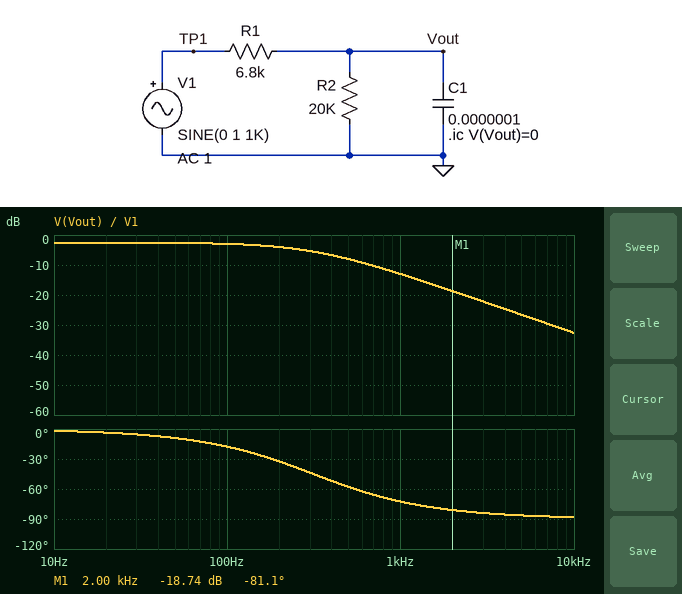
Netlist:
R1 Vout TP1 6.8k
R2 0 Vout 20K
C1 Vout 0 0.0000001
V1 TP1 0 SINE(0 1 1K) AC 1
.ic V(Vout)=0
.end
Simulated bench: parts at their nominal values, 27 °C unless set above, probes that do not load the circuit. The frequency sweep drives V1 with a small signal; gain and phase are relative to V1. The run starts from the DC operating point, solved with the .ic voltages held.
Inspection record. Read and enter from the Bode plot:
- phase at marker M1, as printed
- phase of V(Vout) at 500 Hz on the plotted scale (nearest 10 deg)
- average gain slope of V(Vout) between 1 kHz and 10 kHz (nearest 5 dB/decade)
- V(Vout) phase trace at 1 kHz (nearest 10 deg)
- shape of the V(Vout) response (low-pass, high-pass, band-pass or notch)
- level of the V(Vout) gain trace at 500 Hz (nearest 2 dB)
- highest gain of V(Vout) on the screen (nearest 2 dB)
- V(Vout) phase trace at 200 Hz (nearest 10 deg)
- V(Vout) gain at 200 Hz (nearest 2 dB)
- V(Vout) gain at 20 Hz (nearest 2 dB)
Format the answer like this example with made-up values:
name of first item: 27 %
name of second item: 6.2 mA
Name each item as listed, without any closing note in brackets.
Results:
phase at marker M1, as printed: -81.1 deg
phase of V(Vout) at 500 Hz on the plotted scale: -60 deg
average gain slope of V(Vout) between 1 kHz and 10 kHz: -20 dB/decade
V(Vout) phase trace at 1 kHz: -70 deg
shape of the V(Vout) response: low-pass
level of the V(Vout) gain trace at 500 Hz: -8 dB
highest gain of V(Vout) on the screen: -2 dB
V(Vout) phase trace at 200 Hz: -30 deg
V(Vout) gain at 200 Hz: -4 dB
V(Vout) gain at 20 Hz: -2 dB
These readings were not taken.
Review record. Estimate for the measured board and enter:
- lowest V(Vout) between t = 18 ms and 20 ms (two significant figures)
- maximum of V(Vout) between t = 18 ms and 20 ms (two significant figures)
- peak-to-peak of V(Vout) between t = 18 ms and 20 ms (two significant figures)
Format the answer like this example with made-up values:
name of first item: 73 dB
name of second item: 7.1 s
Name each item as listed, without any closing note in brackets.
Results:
lowest V(Vout) between t = 18 ms and 20 ms: -220 mV
maximum of V(Vout) between t = 18 ms and 20 ms: 220 mV
peak-to-peak of V(Vout) between t = 18 ms and 20 ms: 450 mV
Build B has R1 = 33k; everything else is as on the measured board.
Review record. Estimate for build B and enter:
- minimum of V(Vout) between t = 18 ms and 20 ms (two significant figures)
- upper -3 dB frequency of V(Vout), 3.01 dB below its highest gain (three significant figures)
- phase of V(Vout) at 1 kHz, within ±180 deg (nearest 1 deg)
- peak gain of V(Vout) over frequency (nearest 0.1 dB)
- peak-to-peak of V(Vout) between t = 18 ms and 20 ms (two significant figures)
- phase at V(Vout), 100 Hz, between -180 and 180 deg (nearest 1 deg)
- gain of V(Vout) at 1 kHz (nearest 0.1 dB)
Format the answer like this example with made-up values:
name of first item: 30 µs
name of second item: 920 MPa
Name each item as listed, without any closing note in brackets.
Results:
minimum of V(Vout) between t = 18 ms and 20 ms: -48 mV
upper -3 dB frequency of V(Vout), 3.01 dB below its highest gain: 128 Hz
phase of V(Vout) at 1 kHz, within ±180 deg: -83 deg
peak gain of V(Vout) over frequency: -8.5 dB
peak-to-peak of V(Vout) between t = 18 ms and 20 ms: 96 mV
phase at V(Vout), 100 Hz, between -180 and 180 deg: -38 deg
gain of V(Vout) at 1 kHz: -26.4 dB
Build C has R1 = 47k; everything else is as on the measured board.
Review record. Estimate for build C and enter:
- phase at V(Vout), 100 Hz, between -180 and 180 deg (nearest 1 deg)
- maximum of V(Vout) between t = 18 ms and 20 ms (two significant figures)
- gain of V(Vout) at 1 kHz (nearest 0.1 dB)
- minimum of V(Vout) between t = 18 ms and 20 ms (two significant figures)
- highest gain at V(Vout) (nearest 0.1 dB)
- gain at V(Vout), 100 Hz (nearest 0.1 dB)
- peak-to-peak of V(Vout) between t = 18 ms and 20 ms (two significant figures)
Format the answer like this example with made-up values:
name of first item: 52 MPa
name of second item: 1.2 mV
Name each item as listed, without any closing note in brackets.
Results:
phase at V(Vout), 100 Hz, between -180 and 180 deg: -41 deg
maximum of V(Vout) between t = 18 ms and 20 ms: 34 mV
gain of V(Vout) at 1 kHz: -29.5 dB
minimum of V(Vout) between t = 18 ms and 20 ms: -34 mV
highest gain at V(Vout): -10.5 dB
gain at V(Vout), 100 Hz: -13.0 dB
peak-to-peak of V(Vout) between t = 18 ms and 20 ms: 67 mV
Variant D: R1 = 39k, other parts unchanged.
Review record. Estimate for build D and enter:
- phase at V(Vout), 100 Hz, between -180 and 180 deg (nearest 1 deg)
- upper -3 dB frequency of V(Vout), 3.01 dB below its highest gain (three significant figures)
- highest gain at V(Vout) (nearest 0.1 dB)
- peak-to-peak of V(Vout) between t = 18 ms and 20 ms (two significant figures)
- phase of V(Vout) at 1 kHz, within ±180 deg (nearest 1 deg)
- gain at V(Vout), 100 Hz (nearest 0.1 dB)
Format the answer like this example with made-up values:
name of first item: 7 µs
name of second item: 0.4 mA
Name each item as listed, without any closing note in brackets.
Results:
phase at V(Vout), 100 Hz, between -180 and 180 deg: -40 deg
upper -3 dB frequency of V(Vout), 3.01 dB below its highest gain: 120 Hz
highest gain at V(Vout): -9.4 dB
peak-to-peak of V(Vout) between t = 18 ms and 20 ms: 81 mV
phase of V(Vout) at 1 kHz, within ±180 deg: -83 deg
gain at V(Vout), 100 Hz: -11.7 dB
